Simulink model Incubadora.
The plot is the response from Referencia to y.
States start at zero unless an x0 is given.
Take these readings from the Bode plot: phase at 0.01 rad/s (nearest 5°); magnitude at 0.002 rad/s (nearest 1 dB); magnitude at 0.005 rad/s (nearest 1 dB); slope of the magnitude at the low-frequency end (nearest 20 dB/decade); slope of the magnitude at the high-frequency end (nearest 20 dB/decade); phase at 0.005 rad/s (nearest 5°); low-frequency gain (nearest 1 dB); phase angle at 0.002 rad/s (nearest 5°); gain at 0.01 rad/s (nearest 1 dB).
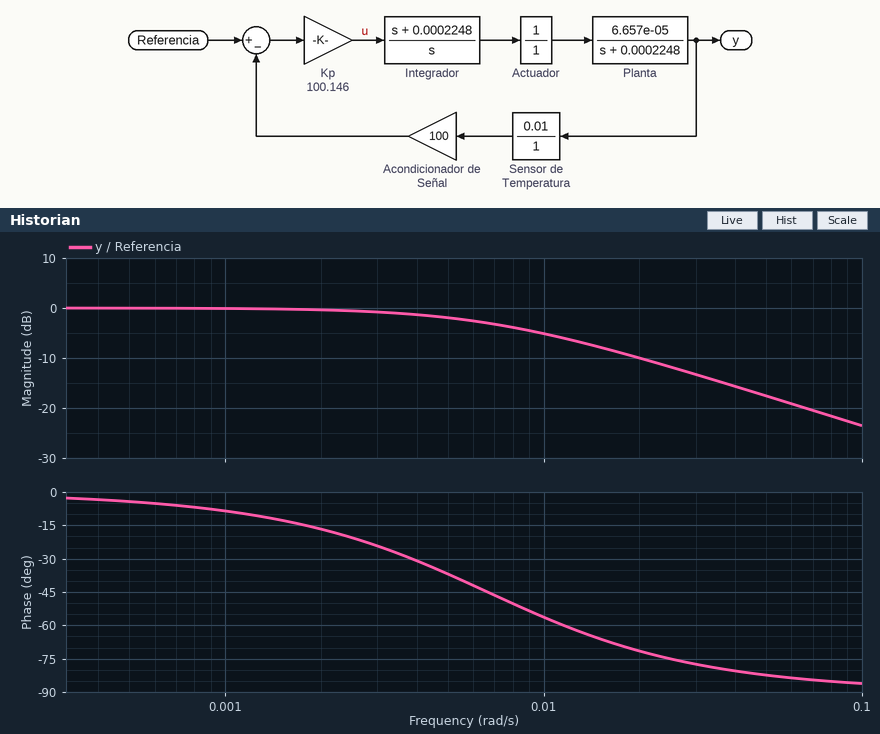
-55°
0 dB
-2 dB
0 dB/decade
-20 dB/decade
-35°
0 dB
-15°
-5 dB
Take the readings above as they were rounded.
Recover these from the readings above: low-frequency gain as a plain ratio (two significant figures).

1.0
